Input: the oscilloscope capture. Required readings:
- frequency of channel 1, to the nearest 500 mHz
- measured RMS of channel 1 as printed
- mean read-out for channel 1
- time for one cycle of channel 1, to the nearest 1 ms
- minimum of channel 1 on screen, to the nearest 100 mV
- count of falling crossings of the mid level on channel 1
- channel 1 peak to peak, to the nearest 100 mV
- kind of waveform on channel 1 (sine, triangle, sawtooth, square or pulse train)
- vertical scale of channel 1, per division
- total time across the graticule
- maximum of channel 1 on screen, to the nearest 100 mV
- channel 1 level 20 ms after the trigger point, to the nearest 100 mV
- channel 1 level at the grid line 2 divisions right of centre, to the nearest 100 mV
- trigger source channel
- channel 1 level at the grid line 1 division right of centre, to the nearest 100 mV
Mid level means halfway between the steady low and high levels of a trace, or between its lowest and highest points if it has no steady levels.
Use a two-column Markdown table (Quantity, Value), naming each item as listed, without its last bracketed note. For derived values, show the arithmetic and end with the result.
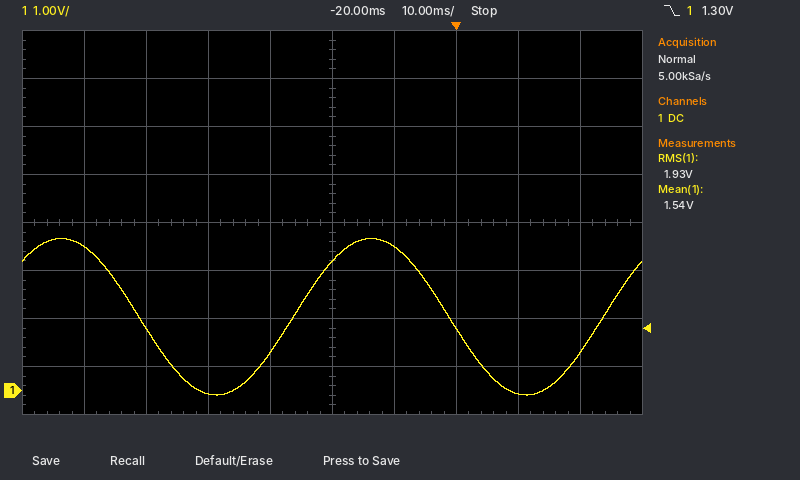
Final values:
| Quantity | Value |
|---|---|
| frequency of channel 1, to the nearest 500 mHz | 1 / 50 ms ≈ 20.0 Hz |
| measured RMS of channel 1 as printed | 1.93 V |
| mean read-out for channel 1 | 1.54 V |
| time for one cycle of channel 1, to the nearest 1 ms | 50 ms |
| minimum of channel 1 on screen, to the nearest 100 mV | -100 mV |
| count of falling crossings of the mid level on channel 1 | 2 |
| channel 1 peak to peak, to the nearest 100 mV | 3.2 V − (-100 mV) = 3.3 V |
| kind of waveform on channel 1 | sine |
| vertical scale of channel 1, per division | 1 V |
| total time across the graticule | 100 ms |
| maximum of channel 1 on screen, to the nearest 100 mV | 3.2 V |
| channel 1 level 20 ms after the trigger point, to the nearest 100 mV | 800 mV |
| channel 1 level at the grid line 2 divisions right of centre, to the nearest 100 mV | 1.3 V |
| trigger source channel | channel 1 |
| channel 1 level at the grid line 1 division right of centre, to the nearest 100 mV | 3.0 V |
